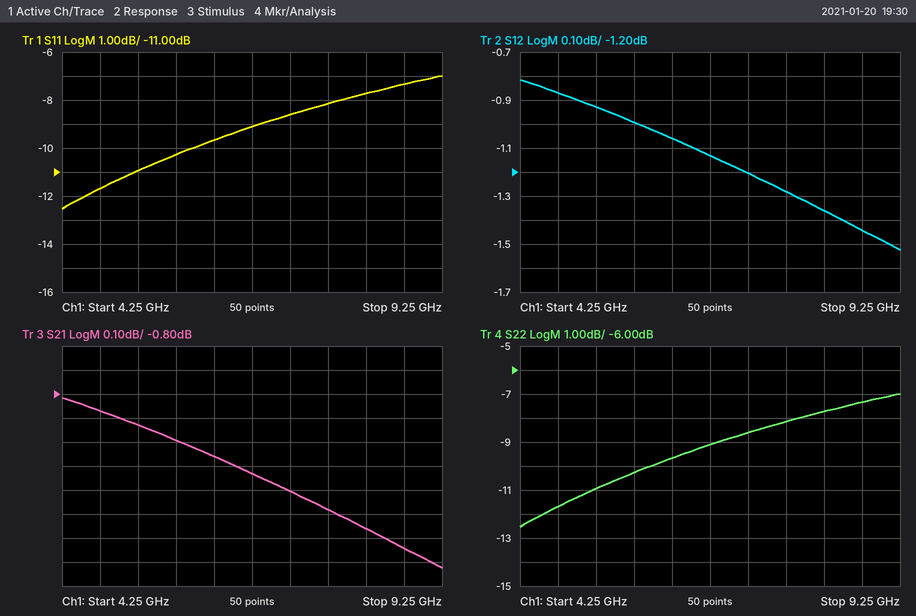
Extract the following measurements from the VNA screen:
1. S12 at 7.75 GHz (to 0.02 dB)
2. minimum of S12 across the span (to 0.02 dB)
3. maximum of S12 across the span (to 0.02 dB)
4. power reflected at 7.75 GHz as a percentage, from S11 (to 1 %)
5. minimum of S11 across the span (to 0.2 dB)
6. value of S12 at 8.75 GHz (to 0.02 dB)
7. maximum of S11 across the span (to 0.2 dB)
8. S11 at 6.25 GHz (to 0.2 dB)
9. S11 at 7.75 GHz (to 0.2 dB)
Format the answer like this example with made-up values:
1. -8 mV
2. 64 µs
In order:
1. -1.28 dB
2. -1.52 dB
3. -0.82 dB
4. 15 %
5. -12.6 dB
6. -1.44 dB
7. -7.0 dB
8. -9.6 dB
9. -8.2 dB
